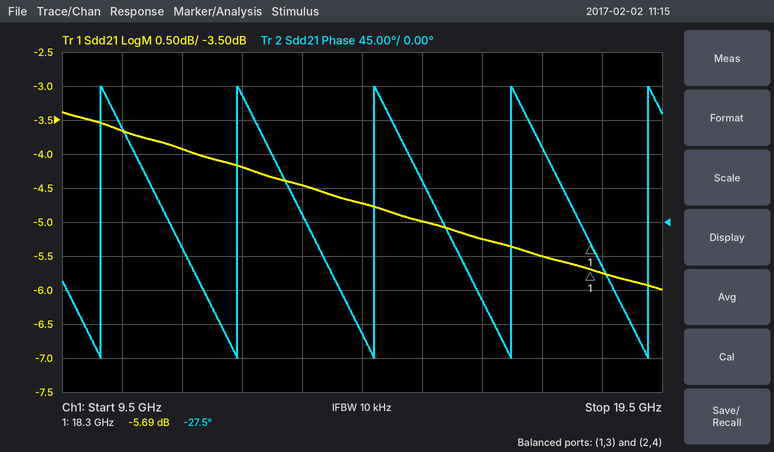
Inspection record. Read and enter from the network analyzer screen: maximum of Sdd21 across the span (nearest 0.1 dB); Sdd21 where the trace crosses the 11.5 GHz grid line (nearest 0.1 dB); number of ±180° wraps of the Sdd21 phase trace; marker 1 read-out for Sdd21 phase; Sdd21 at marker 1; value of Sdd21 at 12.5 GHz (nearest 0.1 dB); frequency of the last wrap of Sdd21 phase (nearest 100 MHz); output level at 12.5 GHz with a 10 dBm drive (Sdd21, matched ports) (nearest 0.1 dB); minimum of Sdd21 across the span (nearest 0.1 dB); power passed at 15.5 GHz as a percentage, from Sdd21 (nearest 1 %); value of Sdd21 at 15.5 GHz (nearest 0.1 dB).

-3.4 dB
-3.9 dB
5
-27.5°
-5.69 dB
-4.2 dB
19.3 GHz
5.8 dBm
-6.0 dB
32 %
-5.0 dB
